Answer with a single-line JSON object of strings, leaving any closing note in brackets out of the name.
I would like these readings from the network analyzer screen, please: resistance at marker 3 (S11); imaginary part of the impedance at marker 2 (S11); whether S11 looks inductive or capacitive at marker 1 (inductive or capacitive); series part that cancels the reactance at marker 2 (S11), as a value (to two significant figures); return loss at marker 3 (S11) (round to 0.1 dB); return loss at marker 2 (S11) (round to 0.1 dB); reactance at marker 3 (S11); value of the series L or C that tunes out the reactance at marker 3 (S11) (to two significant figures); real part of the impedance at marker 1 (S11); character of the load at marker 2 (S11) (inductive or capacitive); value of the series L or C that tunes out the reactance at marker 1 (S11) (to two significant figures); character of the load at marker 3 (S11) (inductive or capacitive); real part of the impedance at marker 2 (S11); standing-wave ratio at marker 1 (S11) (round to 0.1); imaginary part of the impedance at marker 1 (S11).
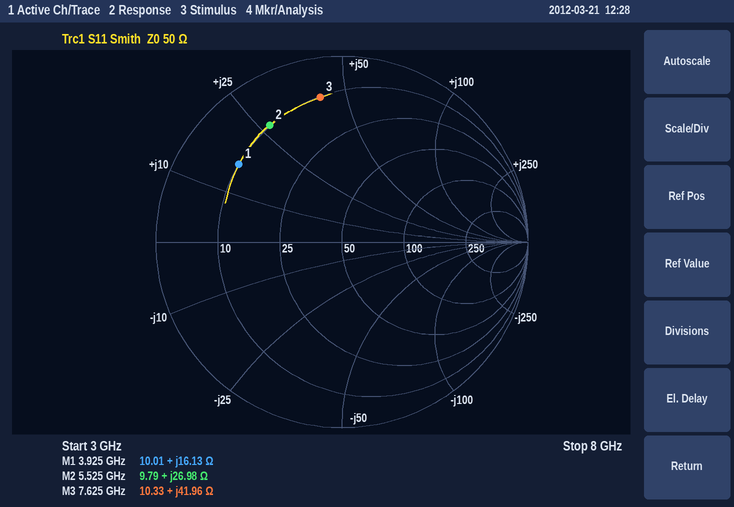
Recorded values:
{"resistance at marker 3": "10.33 Ω", "imaginary part of the impedance at marker 2": "+26.98 Ω", "whether S11 looks inductive or capacitive at marker 1": "inductive", "series part that cancels the reactance at marker 2 (S11), as a value": "1.1 pF", "return loss at marker 3 (S11)": "2.1 dB", "return loss at marker 2 (S11)": "2.6 dB", "reactance at marker 3": "+41.96 Ω", "value of the series L or C that tunes out the reactance at marker 3 (S11)": "500 fF", "real part of the impedance at marker 1": "10.01 Ω", "character of the load at marker 2 (S11)": "inductive", "value of the series L or C that tunes out the reactance at marker 1 (S11)": "2.5 pF", "character of the load at marker 3 (S11)": "inductive", "real part of the impedance at marker 2": "9.79 Ω", "standing-wave ratio at marker 1 (S11)": "5.5", "imaginary part of the impedance at marker 1": "+16.13 Ω"}
